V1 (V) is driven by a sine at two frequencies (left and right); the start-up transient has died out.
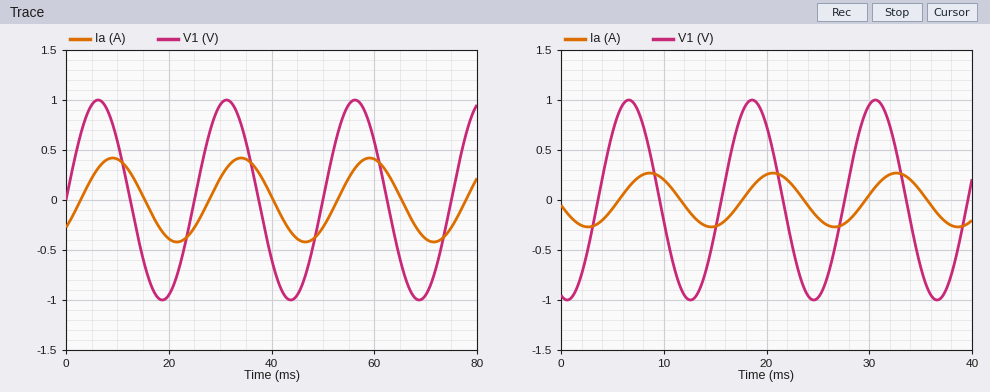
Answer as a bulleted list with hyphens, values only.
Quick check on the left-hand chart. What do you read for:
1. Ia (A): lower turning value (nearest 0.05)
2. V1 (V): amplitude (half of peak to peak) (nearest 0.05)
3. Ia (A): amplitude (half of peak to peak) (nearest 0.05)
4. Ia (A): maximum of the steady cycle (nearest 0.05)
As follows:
- -0.40
- 1.00
- 0.40
- 0.40
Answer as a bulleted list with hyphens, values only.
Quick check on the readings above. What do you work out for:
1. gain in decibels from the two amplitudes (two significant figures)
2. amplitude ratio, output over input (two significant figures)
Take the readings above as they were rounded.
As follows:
- -8.0 dB
- 0.40
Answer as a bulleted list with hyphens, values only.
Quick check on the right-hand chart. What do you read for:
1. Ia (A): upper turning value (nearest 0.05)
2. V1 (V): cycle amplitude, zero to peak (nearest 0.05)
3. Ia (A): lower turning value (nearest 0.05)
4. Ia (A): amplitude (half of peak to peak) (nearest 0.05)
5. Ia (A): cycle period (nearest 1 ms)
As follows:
- 0.25
- 1.00
- -0.25
- 0.25
- 12 ms
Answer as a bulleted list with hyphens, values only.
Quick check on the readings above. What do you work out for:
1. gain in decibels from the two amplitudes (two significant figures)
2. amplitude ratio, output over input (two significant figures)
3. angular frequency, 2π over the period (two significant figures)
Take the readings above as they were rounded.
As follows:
- -12 dB
- 0.25
- 0.52 rad/ms
